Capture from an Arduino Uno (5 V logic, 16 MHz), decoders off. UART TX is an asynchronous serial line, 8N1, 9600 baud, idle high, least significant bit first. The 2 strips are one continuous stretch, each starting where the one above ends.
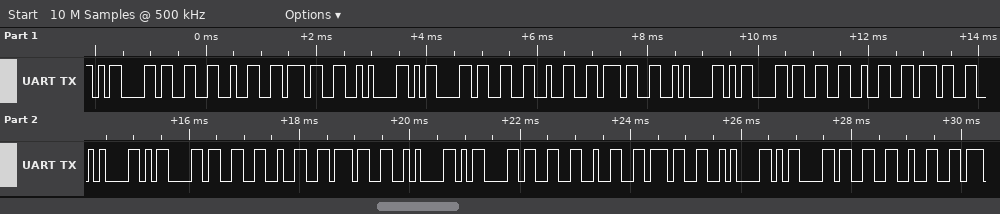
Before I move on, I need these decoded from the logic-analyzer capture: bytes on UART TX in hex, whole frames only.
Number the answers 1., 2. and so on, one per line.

1. 0D 33 32 37 0A 0D 33 32 37 0A 0D 33 32 37 0A 0D 33 32 37 0A 0D 33 32 37 0A 0D 33 32
